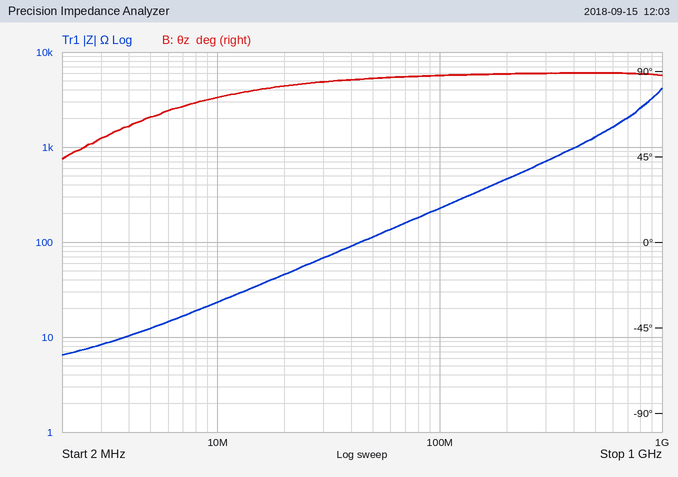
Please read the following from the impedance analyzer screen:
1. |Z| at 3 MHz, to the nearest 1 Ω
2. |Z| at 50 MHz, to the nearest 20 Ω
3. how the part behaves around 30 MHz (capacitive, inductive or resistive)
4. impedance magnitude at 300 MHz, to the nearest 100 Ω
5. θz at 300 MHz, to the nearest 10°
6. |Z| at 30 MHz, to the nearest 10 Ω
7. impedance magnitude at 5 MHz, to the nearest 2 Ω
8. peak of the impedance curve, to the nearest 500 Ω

8 Ω
120 Ω
inductive
700 Ω
90°
70 Ω
12 Ω
4.0 kΩ
